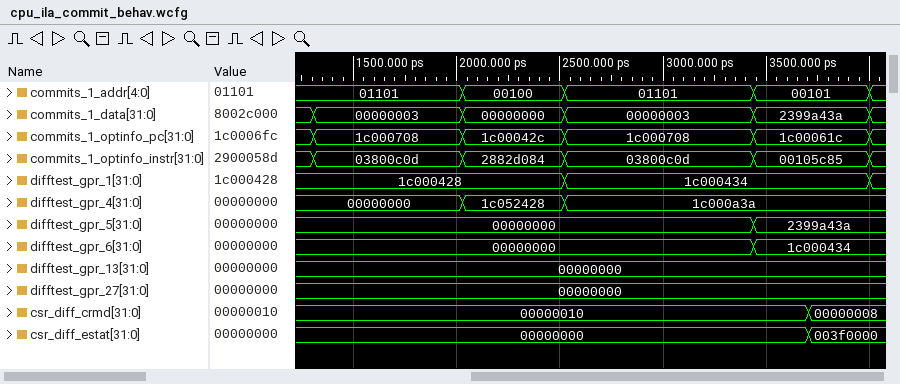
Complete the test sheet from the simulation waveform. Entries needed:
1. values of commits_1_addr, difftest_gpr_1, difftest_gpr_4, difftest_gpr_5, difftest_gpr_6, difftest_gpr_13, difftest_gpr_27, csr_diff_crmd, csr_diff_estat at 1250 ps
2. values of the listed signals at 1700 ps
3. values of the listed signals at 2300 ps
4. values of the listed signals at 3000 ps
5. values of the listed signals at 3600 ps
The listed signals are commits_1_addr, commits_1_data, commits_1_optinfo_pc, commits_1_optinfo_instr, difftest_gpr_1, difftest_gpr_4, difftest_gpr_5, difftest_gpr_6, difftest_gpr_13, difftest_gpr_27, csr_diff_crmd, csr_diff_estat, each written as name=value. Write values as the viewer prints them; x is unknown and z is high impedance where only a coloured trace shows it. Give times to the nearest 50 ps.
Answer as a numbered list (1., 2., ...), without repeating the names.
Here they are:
1. commits_1_addr=01101, difftest_gpr_1=1c000428, difftest_gpr_4=00000000, difftest_gpr_5=00000000, difftest_gpr_6=00000000, difftest_gpr_13=00000000, difftest_gpr_27=00000000, csr_diff_crmd=00000010, csr_diff_estat=00000000
2. commits_1_addr=01101, commits_1_data=00000003, commits_1_optinfo_pc=1c000708, commits_1_optinfo_instr=03800c0d, difftest_gpr_1=1c000428, difftest_gpr_4=00000000, difftest_gpr_5=00000000, difftest_gpr_6=00000000, difftest_gpr_13=00000000, difftest_gpr_27=00000000, csr_diff_crmd=00000010, csr_diff_estat=00000000
3. commits_1_addr=00100, commits_1_data=00000000, commits_1_optinfo_pc=1c00042c, commits_1_optinfo_instr=2882d084, difftest_gpr_1=1c000428, difftest_gpr_4=1c052428, difftest_gpr_5=00000000, difftest_gpr_6=00000000, difftest_gpr_13=00000000, difftest_gpr_27=00000000, csr_diff_crmd=00000010, csr_diff_estat=00000000
4. commits_1_addr=01101, commits_1_data=00000003, commits_1_optinfo_pc=1c000708, commits_1_optinfo_instr=03800c0d, difftest_gpr_1=1c000434, difftest_gpr_4=1c000a3a, difftest_gpr_5=00000000, difftest_gpr_6=00000000, difftest_gpr_13=00000000, difftest_gpr_27=00000000, csr_diff_crmd=00000010, csr_diff_estat=00000000
5. commits_1_addr=00101, commits_1_data=2399a43a, commits_1_optinfo_pc=1c00061c, commits_1_optinfo_instr=00105c85, difftest_gpr_1=1c000434, difftest_gpr_4=1c000a3a, difftest_gpr_5=2399a43a, difftest_gpr_6=1c000434, difftest_gpr_13=00000000, difftest_gpr_27=00000000, csr_diff_crmd=00000010, csr_diff_estat=00000000
